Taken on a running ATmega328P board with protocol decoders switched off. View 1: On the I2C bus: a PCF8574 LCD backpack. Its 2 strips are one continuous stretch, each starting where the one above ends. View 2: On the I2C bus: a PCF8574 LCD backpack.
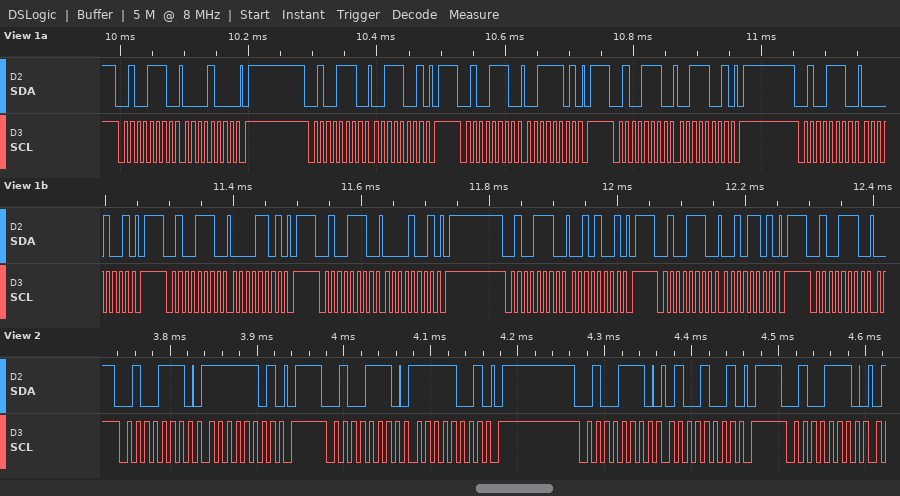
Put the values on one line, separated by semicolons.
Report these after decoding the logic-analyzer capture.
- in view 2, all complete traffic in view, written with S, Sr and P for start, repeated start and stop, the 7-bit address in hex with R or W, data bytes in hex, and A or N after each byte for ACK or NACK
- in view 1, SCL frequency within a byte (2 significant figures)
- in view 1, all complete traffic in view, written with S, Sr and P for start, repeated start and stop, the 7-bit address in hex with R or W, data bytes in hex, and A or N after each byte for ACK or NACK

S 27W A FD A P S 27W A F9 A P S 27W A 49 A P S 27W A; 100 kHz; S 27W A 08 A P S 27W A 39 A P S 27W A 3D A P S 27W A 39 A P S 27W A 09 A P S 27W A 0D A P S 27W A 09 A P S 27W A 29 A P S 27W A 2D A P S 27W A
